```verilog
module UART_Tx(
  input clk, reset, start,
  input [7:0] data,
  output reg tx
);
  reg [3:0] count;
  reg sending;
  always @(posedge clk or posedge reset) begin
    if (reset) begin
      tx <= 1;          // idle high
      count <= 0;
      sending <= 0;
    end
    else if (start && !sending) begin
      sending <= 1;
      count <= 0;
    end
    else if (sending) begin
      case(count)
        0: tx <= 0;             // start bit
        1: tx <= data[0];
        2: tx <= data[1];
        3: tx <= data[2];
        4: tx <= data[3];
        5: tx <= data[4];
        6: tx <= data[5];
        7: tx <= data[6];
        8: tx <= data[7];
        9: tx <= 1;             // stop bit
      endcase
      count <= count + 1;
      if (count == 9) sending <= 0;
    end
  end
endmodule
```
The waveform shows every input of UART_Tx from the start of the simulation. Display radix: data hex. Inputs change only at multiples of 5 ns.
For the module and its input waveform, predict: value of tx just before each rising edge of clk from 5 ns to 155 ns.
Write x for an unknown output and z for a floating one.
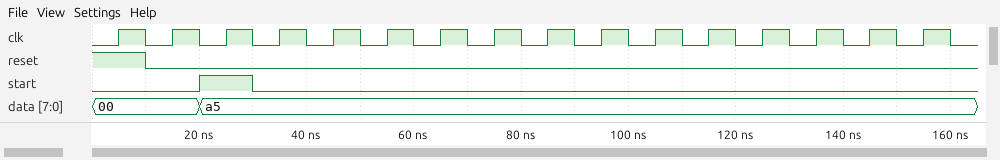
1 1 1 1 0 1 0 1 0 0 1 0 1 1 1 1
